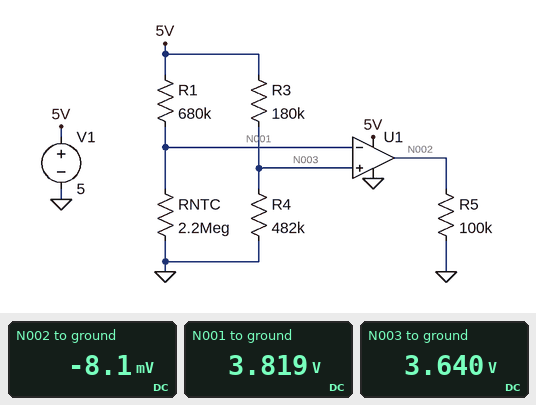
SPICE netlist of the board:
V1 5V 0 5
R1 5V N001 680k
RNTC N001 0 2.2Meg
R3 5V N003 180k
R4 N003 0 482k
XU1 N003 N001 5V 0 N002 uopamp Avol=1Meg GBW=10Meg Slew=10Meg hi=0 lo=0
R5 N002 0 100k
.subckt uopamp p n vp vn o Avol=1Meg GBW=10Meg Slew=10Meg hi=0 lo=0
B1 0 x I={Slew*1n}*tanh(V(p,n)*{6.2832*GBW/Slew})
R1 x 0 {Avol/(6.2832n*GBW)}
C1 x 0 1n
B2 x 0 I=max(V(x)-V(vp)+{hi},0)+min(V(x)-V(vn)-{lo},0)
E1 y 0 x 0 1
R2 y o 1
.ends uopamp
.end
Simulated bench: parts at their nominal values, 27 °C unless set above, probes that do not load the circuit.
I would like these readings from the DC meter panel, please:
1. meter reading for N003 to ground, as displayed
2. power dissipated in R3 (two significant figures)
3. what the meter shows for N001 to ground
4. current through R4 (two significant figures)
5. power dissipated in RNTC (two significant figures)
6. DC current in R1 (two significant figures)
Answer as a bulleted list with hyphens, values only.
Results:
- 3.640 V
- 10 µW
- 3.819 V
- 7.6 µA
- 6.6 µW
- 1.7 µA
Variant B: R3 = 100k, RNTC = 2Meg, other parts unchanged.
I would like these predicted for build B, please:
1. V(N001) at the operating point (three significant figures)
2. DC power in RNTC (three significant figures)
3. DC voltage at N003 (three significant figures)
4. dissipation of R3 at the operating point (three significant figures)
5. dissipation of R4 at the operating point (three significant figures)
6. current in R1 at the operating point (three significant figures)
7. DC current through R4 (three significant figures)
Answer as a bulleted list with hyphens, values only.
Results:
- 3.73 V
- 6.96 µW
- 4.14 V
- 7.38 µW
- 35.6 µW
- 1.87 µA
- 8.59 µA
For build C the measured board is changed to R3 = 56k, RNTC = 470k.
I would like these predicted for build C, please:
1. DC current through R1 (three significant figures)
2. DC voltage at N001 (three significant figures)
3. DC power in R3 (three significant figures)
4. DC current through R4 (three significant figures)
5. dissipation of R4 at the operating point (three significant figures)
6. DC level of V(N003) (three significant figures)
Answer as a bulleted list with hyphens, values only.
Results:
- 4.35 µA
- 2.04 V
- 4.84 µW
- 9.29 µA
- 41.6 µW
- 4.48 V
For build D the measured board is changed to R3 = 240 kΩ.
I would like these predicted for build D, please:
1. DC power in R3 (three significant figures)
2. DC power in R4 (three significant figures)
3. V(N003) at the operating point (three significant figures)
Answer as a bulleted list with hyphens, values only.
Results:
- 11.5 µW
- 23.1 µW
- 3.34 V
